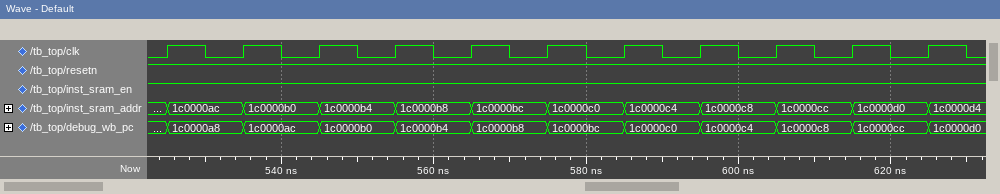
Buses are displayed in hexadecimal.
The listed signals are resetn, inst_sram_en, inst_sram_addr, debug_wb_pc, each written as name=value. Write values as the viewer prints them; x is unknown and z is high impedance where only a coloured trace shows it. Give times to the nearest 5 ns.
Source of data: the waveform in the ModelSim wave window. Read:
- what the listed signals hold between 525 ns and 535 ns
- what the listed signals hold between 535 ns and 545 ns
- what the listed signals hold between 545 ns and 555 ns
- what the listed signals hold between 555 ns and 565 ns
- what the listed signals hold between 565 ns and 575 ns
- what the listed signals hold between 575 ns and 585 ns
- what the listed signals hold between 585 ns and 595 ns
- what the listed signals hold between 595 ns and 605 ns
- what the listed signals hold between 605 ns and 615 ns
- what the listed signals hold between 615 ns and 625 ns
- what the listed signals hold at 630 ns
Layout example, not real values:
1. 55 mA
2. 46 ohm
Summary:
1. resetn=1, inst_sram_en=1, inst_sram_addr=1c0000ac, debug_wb_pc=1c0000a8
2. resetn=1, inst_sram_en=1, inst_sram_addr=1c0000b0, debug_wb_pc=1c0000ac
3. resetn=1, inst_sram_en=1, inst_sram_addr=1c0000b4, debug_wb_pc=1c0000b0
4. resetn=1, inst_sram_en=1, inst_sram_addr=1c0000b8, debug_wb_pc=1c0000b4
5. resetn=1, inst_sram_en=1, inst_sram_addr=1c0000bc, debug_wb_pc=1c0000b8
6. resetn=1, inst_sram_en=1, inst_sram_addr=1c0000c0, debug_wb_pc=1c0000bc
7. resetn=1, inst_sram_en=1, inst_sram_addr=1c0000c4, debug_wb_pc=1c0000c0
8. resetn=1, inst_sram_en=1, inst_sram_addr=1c0000c8, debug_wb_pc=1c0000c4
9. resetn=1, inst_sram_en=1, inst_sram_addr=1c0000cc, debug_wb_pc=1c0000c8
10. resetn=1, inst_sram_en=1, inst_sram_addr=1c0000d0, debug_wb_pc=1c0000cc
11. resetn=1, inst_sram_en=1, inst_sram_addr=1c0000d4, debug_wb_pc=1c0000d0
